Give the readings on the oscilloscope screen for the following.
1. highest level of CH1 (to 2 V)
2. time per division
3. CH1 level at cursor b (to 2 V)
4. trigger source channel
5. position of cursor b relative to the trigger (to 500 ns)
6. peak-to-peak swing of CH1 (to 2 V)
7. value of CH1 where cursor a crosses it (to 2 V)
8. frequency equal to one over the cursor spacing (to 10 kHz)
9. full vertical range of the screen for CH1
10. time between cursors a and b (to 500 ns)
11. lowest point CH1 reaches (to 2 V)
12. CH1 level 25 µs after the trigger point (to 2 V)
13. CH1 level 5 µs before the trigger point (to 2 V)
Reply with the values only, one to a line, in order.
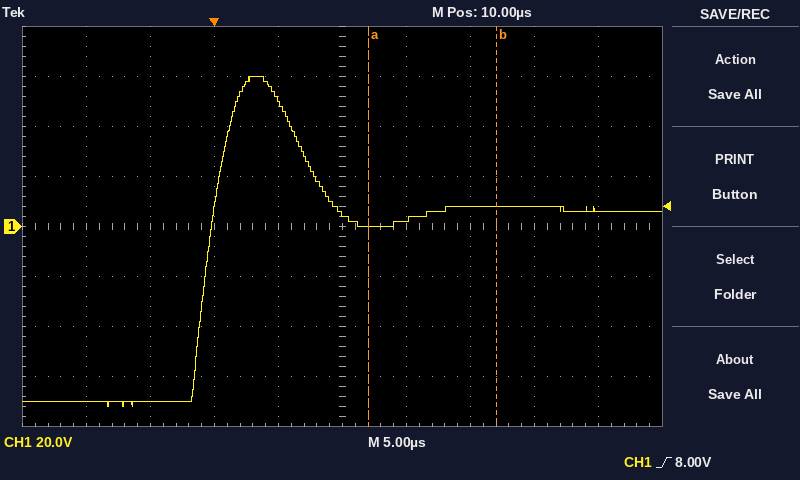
60 V
5 µs
8 V
CH1
+22.0 µs
132 V
0 V
100 kHz
160 V
10.0 µs
-72 V
8 V
-70 V
